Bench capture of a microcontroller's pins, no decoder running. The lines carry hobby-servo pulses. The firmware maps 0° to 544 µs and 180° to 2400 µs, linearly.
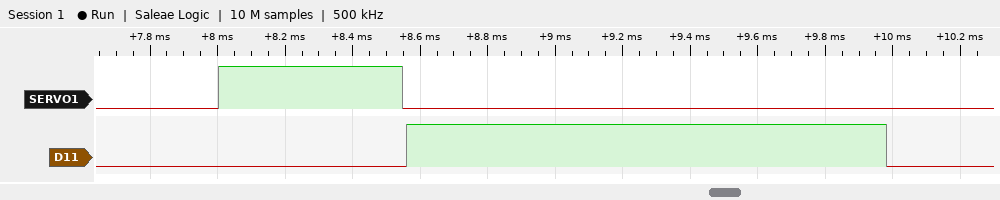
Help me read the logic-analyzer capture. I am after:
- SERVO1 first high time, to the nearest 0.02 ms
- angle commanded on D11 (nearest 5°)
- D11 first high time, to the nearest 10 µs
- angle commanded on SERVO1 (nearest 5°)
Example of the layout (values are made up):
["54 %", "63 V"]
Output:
["0.54 ms", "85°", "1420 µs", "0°"]
